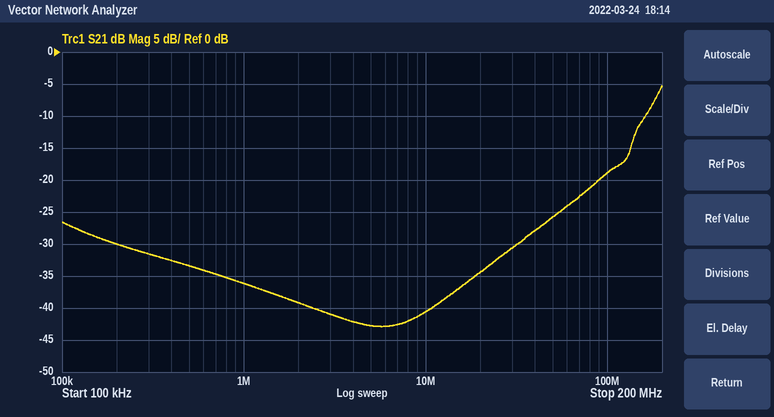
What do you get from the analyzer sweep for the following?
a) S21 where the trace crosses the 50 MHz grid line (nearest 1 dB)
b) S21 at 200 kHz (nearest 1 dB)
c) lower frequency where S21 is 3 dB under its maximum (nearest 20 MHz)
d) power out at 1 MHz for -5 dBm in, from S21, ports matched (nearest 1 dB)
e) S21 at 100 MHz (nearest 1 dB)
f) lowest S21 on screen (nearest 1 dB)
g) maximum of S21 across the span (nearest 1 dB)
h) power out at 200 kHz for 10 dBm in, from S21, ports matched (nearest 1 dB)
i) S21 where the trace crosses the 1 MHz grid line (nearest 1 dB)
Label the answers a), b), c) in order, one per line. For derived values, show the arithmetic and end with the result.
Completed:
a) -26 dB
b) -30 dB
c) 180 MHz
d) -5 dBm + (-36 dB) = -41 dBm
e) -19 dB
f) -43 dB
g) -5 dB
h) 10 dBm + (-30 dB) = -20 dBm
i) -36 dB
